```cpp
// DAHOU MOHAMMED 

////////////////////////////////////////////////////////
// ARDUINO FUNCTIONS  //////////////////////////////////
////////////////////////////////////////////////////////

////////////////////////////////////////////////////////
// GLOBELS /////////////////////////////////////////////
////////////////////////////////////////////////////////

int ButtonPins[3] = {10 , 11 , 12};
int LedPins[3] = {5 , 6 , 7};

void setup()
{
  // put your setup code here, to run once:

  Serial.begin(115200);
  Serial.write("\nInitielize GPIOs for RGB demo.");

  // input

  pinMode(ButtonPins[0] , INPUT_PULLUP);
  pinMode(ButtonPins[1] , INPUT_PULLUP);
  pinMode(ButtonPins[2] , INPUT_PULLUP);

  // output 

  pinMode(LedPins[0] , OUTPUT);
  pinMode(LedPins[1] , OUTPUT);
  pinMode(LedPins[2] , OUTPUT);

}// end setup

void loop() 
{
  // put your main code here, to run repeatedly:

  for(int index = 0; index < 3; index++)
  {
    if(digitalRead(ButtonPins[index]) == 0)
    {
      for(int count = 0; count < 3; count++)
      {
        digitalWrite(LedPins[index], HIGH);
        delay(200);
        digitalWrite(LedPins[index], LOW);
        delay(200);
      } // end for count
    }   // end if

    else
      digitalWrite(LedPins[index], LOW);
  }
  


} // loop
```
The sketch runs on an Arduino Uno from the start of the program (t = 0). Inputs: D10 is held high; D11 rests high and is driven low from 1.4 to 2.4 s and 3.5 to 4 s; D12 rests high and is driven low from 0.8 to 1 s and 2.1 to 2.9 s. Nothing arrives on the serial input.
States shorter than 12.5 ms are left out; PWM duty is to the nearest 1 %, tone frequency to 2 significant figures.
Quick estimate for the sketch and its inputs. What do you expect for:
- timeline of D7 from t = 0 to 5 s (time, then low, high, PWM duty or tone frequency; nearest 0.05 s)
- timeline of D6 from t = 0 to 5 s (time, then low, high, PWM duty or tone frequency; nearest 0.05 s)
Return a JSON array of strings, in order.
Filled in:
["0 s low; 0.8 s high; 1 s low; 1.2 s high; 1.4 s low; 1.6 s high; 1.8 s low", "0 s low; 2 s high; 2.2 s low; 2.4 s high; 2.6 s low; 2.8 s high; 3 s low; 3.5 s high; 3.7 s low; 3.9 s high; 4.1 s low; 4.3 s high; 4.5 s low"]
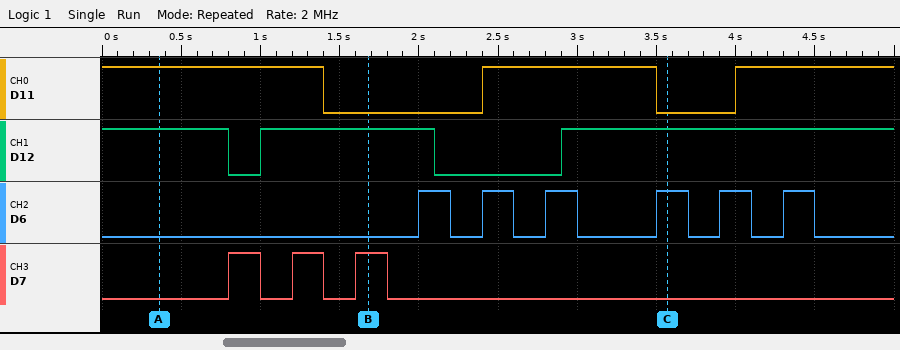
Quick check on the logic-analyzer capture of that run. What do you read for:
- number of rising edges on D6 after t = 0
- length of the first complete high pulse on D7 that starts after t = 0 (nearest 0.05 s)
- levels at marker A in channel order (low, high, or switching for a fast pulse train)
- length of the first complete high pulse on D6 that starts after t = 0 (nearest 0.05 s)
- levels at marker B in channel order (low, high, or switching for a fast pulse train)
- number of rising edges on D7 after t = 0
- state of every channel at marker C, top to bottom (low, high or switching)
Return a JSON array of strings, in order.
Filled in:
["6", "0.20 s", "D11 high, D12 high, D6 low, D7 low", "0.20 s", "D11 low, D12 high, D6 low, D7 high", "3", "D11 low, D12 high, D6 high, D7 low"]
